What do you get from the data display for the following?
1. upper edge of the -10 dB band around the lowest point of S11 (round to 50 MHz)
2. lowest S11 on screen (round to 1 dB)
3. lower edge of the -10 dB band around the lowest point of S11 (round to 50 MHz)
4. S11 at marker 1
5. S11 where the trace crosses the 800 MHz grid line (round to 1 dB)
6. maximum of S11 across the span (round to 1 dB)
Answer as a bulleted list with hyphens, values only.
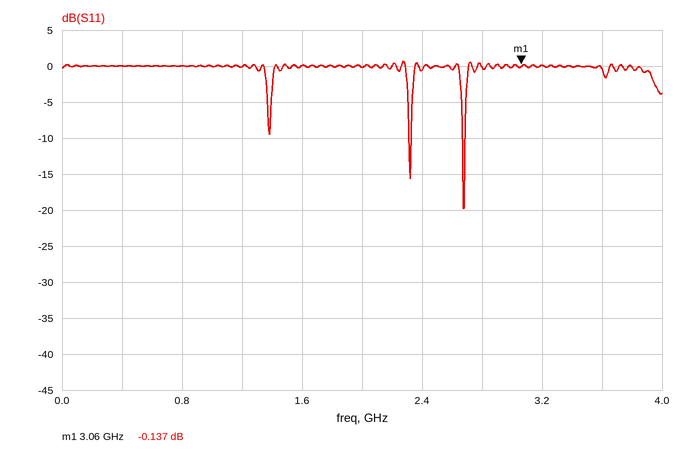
- 2.70 GHz
- -20 dB
- 2.65 GHz
- -0.137 dB
- 0 dB
- 1 dB
